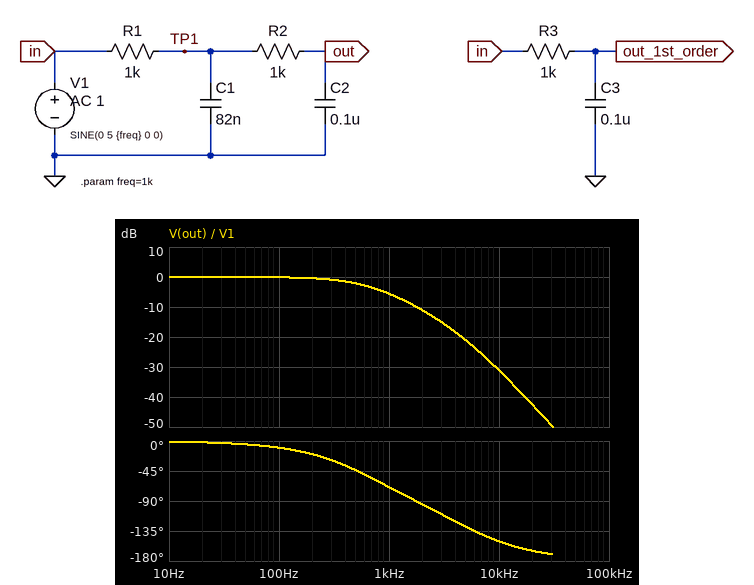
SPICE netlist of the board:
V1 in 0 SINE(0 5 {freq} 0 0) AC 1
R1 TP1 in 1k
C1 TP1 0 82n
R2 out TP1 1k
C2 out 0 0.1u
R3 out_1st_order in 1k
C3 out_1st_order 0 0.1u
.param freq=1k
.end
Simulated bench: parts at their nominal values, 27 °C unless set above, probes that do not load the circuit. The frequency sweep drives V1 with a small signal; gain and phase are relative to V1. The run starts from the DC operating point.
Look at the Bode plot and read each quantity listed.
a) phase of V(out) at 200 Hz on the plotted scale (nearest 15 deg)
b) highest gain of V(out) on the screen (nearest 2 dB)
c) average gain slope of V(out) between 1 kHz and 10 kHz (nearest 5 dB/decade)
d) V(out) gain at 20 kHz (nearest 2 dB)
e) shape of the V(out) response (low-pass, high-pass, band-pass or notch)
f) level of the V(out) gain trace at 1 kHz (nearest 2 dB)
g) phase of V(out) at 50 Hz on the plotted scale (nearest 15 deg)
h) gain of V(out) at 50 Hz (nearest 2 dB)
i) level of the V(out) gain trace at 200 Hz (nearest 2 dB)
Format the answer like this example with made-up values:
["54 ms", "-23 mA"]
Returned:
["-15 deg", "0 dB", "-25 dB/decade", "-42 dB", "low-pass", "-6 dB", "0 deg", "0 dB", "0 dB"]
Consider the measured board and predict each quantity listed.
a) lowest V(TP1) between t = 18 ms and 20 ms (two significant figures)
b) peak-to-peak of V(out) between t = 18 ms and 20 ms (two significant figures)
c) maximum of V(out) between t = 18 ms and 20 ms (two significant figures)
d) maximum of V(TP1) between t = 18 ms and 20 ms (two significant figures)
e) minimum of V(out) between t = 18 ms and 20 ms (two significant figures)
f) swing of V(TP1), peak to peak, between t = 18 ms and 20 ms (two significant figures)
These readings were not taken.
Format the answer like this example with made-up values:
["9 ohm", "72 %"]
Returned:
["-3.1 V", "5.3 V", "2.6 V", "3.1 V", "-2.6 V", "6.2 V"]
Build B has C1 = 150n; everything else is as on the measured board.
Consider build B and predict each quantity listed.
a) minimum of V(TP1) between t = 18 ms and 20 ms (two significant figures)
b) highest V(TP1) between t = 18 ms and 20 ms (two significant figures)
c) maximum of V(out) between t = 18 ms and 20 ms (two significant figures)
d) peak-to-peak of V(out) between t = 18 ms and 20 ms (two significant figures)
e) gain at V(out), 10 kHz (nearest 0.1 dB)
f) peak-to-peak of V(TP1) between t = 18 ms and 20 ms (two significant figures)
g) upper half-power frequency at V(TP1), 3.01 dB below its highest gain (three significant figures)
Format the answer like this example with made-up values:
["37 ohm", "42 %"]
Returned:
["-2.6 V", "2.6 V", "2.2 V", "4.5 V", "-35.9 dB", "5.3 V", "579 Hz"]
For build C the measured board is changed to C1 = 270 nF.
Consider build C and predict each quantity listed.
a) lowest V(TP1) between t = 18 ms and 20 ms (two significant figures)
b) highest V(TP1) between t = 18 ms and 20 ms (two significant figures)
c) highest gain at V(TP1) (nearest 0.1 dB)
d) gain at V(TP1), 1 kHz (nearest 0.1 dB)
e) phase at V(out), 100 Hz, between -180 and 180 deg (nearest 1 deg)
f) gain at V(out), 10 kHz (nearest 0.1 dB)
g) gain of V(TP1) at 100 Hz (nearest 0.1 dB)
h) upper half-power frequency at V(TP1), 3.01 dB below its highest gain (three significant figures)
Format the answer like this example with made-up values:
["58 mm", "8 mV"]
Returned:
["-2.0 V", "2.0 V", "0 dB", "-8.0 dB", "-17 deg", "-40.8 dB", "-0.3 dB", "409 Hz"]
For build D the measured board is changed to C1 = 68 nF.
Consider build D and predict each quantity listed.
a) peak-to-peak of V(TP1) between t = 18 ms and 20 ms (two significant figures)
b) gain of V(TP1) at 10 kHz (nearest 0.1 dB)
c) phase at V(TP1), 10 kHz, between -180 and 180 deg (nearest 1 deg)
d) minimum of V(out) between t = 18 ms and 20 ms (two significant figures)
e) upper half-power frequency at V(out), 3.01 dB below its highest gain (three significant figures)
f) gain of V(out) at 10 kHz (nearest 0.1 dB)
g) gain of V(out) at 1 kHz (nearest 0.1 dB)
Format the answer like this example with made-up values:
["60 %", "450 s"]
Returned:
["6.4 V", "-13.7 dB", "-66 deg", "-2.7 V", "655 Hz", "-29.8 dB", "-5.3 dB"]
